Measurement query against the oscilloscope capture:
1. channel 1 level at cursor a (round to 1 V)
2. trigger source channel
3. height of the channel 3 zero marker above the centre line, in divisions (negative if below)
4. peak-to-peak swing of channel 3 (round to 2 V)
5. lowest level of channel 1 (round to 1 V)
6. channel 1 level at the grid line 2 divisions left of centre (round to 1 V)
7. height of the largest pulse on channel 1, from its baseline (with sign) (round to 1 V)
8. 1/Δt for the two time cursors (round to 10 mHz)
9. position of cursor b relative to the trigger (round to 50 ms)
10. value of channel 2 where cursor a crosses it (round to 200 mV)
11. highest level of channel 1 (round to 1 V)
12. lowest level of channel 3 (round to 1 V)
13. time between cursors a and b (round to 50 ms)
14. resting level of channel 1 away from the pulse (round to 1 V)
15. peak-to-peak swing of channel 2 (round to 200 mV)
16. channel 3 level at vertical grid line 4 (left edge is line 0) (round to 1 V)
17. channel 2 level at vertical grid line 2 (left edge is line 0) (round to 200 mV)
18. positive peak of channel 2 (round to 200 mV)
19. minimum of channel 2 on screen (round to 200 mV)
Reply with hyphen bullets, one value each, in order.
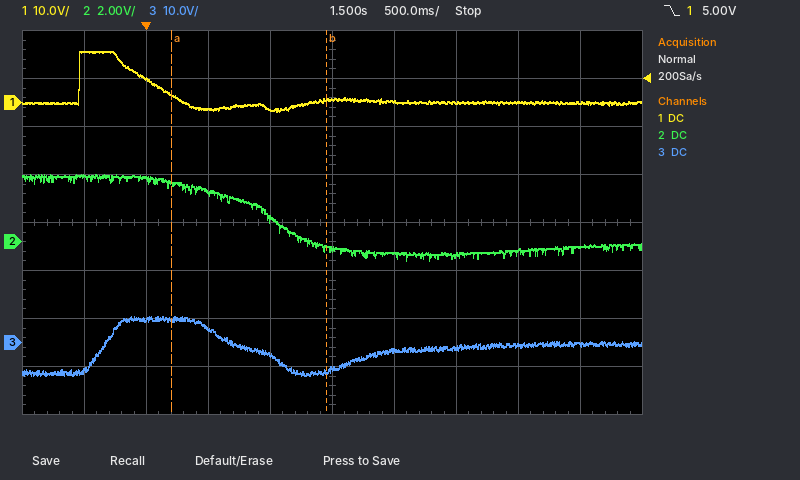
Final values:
- 2 V
- channel 1
- -2.5 div
- 12 V
- -2 V
- -1 V
- +11 V
- 800 mHz
- +1.45 s
- 2.4 V
- 11 V
- -7 V
- 1.25 s
- 0 V
- 3.6 V
- -3 V
- 2.6 V
- 2.8 V
- -800 mV
